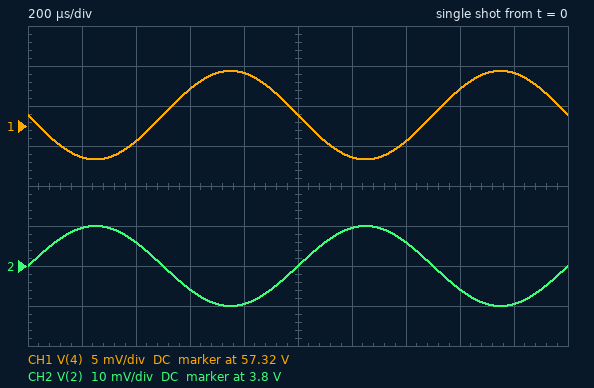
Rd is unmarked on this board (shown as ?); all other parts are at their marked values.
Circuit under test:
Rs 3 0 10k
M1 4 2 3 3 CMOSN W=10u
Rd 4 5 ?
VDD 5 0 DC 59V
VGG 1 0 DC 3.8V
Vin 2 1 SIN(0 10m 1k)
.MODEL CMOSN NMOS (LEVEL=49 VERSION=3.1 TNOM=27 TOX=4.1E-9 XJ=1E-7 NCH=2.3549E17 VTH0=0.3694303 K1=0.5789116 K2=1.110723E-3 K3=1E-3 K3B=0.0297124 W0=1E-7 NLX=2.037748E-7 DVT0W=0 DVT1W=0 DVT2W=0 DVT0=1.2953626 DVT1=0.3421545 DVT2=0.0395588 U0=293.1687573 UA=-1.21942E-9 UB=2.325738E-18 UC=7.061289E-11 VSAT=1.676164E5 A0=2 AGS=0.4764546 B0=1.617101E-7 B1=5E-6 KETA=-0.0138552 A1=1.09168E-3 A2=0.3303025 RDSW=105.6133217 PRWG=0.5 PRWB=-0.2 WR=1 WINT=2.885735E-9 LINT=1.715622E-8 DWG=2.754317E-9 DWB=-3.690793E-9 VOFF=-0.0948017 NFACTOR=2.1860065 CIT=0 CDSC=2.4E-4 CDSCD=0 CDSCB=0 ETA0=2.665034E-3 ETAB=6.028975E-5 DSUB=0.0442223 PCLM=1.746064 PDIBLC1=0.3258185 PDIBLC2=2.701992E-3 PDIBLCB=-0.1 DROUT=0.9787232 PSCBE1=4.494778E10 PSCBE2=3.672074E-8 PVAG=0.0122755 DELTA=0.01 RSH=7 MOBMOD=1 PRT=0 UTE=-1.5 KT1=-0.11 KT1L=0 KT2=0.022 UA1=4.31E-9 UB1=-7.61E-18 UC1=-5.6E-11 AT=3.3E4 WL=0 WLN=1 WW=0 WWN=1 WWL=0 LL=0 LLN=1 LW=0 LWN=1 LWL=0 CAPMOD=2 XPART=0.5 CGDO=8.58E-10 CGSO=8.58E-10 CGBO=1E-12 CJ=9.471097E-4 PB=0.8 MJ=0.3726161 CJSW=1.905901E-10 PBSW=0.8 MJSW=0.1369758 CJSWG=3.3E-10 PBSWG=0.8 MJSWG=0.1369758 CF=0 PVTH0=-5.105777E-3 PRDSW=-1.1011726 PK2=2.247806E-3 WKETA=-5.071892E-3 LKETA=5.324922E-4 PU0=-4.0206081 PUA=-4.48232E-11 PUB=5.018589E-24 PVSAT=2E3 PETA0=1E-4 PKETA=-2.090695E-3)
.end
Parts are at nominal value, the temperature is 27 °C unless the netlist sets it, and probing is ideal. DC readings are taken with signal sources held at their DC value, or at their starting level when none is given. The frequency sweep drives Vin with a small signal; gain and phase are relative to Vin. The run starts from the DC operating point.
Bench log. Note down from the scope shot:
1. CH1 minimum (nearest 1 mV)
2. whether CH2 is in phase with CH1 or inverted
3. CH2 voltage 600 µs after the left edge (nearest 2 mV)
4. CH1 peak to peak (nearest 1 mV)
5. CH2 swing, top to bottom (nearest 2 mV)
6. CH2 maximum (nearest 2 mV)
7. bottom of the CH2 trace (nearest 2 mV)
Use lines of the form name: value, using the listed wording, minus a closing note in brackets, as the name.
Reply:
CH1 minimum: 57.316 V
whether CH2 is in phase with CH1 or inverted: inverted
CH2 voltage 600 µs after the left edge: 3.794 V
CH1 peak to peak: 11 mV
CH2 swing, top to bottom: 20 mV
CH2 maximum: 3.810 V
bottom of the CH2 trace: 3.790 V
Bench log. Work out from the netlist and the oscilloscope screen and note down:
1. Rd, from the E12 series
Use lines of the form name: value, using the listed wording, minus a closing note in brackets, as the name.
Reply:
Rd, from the E12 series: 6.8 kΩ
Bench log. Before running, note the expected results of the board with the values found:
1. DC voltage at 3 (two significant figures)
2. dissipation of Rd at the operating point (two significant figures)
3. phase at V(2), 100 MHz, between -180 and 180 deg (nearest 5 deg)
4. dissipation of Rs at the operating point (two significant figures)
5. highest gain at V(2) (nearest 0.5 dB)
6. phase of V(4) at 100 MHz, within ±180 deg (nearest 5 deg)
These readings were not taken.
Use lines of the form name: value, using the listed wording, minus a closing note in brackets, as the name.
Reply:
DC voltage at 3: 2.5 V
dissipation of Rd at the operating point: 410 µW
phase at V(2), 100 MHz, between -180 and 180 deg: 0 deg
dissipation of Rs at the operating point: 610 µW
highest gain at V(2): 0 dB
phase of V(4) at 100 MHz, within ±180 deg: 150 deg
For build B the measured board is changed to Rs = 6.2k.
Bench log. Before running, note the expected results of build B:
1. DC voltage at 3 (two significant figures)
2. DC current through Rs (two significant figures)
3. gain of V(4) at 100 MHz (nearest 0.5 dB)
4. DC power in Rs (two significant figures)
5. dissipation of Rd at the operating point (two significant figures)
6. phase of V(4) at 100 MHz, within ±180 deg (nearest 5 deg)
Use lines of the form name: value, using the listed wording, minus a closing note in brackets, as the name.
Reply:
DC voltage at 3: 2.2 V
DC current through Rs: 360 µA
gain of V(4) at 100 MHz: -1.5 dB
DC power in Rs: 800 µW
dissipation of Rd at the operating point: 880 µW
phase of V(4) at 100 MHz, within ±180 deg: 155 deg
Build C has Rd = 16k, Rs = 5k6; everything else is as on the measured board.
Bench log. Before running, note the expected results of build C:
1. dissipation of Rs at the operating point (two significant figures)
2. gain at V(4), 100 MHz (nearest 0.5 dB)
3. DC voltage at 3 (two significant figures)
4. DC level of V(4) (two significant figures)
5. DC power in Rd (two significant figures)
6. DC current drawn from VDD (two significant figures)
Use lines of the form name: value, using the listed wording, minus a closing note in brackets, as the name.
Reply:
dissipation of Rs at the operating point: 840 µW
gain at V(4), 100 MHz: 6.5 dB
DC voltage at 3: 2.2 V
DC level of V(4): 53 V
DC power in Rd: 2.4 mW
DC current drawn from VDD: 390 µA
